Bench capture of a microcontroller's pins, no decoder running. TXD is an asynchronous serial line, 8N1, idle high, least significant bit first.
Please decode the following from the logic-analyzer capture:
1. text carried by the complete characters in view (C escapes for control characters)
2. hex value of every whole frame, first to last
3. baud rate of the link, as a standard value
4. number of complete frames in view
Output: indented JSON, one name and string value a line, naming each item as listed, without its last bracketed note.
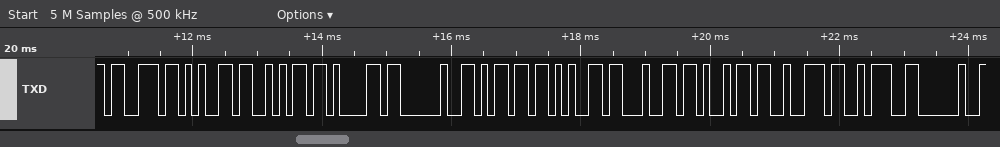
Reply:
{
  "text carried by the complete characters in view": "\"seja medir: \"",
  "hex value of every whole frame, first to last": "0x73 0x65 0x6A 0x61 0x20 0x6D 0x65 0x64 0x69 0x72 0x3A 0x20",
  "baud rate of the link, as a standard value": "9600 baud",
  "number of complete frames in view": "12"
}
